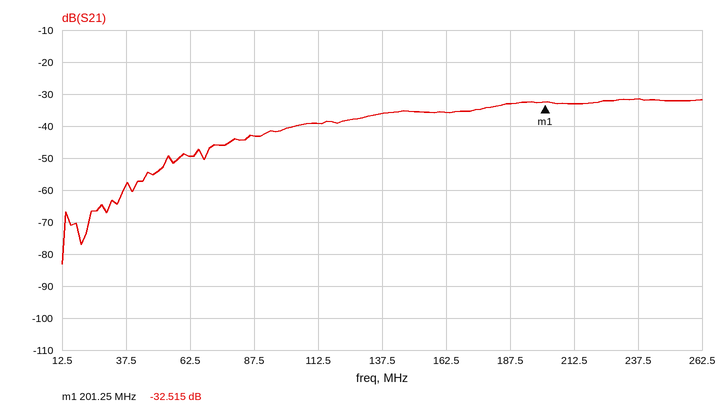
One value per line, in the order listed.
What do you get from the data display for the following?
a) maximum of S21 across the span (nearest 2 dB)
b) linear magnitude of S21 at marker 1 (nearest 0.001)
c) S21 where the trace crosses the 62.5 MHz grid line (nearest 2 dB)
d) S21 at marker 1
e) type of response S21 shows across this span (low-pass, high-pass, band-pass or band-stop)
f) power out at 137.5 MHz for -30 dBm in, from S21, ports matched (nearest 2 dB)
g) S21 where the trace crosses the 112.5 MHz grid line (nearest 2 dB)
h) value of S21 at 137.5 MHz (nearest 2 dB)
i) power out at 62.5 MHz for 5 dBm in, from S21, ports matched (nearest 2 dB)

-32 dB
0.024
-50 dB
-32.515 dB
high-pass
-66 dBm
-40 dB
-36 dB
-44 dBm
